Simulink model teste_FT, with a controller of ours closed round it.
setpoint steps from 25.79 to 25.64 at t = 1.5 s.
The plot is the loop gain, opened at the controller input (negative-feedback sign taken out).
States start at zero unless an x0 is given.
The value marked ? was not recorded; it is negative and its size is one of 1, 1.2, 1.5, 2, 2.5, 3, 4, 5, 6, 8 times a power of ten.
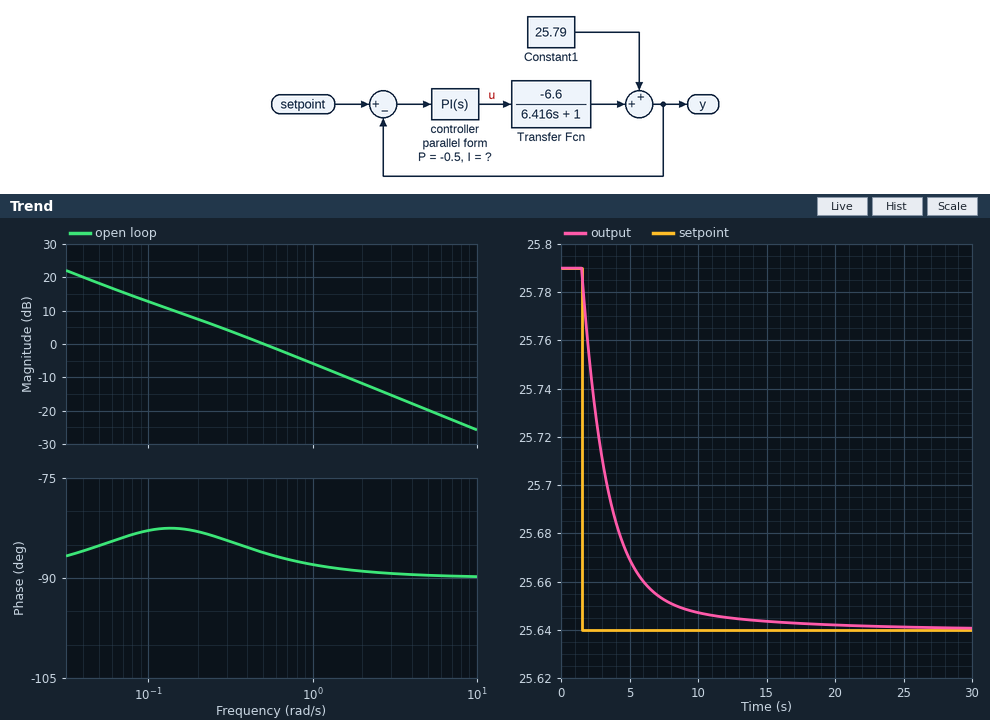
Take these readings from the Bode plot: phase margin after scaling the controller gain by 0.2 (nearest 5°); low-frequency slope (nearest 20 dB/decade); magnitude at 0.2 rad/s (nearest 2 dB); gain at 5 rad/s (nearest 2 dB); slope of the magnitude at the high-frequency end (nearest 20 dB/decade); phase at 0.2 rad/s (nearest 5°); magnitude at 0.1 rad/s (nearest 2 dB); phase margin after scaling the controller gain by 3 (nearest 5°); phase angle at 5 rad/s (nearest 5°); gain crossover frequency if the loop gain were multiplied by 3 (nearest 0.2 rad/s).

95°
-20 dB/decade
8 dB
-20 dB
-20 dB/decade
-85°
12 dB
90°
-90°
1.6 rad/s
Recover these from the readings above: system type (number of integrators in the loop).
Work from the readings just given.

1
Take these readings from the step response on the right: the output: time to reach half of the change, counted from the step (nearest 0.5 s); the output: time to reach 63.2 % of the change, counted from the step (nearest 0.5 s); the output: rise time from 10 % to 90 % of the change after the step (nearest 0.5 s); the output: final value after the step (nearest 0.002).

1.5 s
2.0 s
5.0 s
25.640
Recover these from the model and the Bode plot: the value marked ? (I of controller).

-0.06
